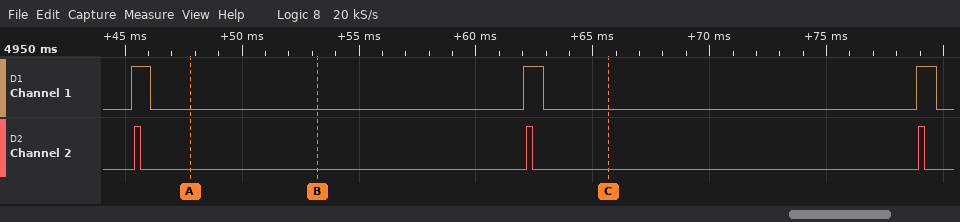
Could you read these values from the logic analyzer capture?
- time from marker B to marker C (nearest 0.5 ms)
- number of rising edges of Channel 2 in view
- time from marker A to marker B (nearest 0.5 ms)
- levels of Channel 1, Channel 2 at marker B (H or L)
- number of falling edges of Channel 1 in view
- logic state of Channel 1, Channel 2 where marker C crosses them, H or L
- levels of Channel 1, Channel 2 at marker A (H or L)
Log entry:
12.5 ms
3
5.5 ms
Channel 1=L, Channel 2=L
3
Channel 1=L, Channel 2=L
Channel 1=L, Channel 2=L
